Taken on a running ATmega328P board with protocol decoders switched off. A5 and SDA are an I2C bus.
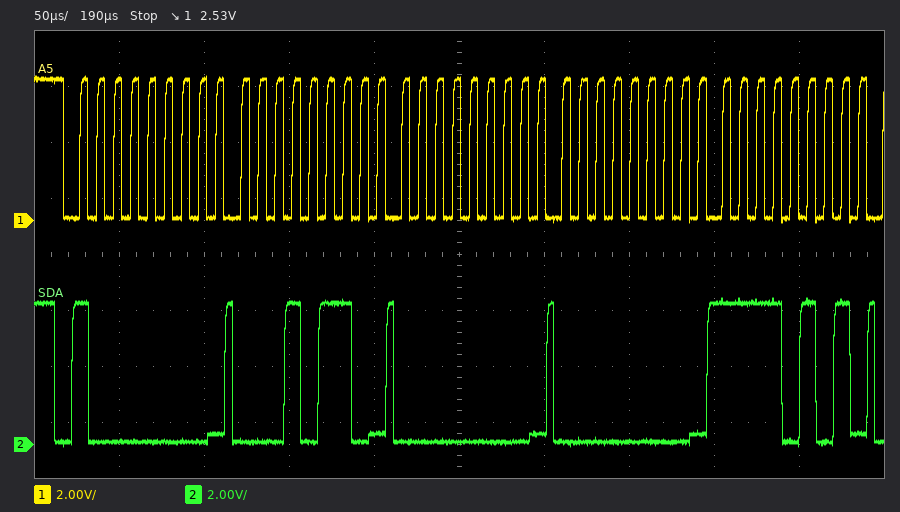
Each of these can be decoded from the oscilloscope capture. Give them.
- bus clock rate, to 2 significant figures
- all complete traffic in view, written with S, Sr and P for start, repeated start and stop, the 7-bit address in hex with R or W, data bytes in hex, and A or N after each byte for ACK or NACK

100 kHz
S 40W A 16 A 00 A 00 A F5 A
